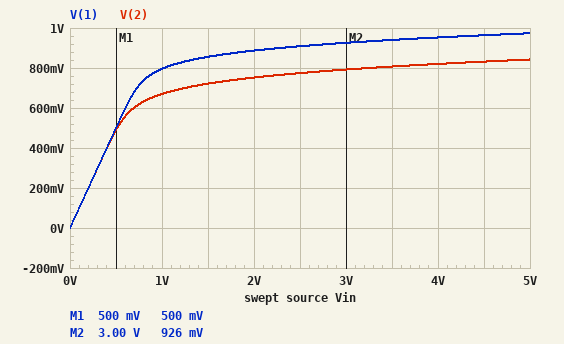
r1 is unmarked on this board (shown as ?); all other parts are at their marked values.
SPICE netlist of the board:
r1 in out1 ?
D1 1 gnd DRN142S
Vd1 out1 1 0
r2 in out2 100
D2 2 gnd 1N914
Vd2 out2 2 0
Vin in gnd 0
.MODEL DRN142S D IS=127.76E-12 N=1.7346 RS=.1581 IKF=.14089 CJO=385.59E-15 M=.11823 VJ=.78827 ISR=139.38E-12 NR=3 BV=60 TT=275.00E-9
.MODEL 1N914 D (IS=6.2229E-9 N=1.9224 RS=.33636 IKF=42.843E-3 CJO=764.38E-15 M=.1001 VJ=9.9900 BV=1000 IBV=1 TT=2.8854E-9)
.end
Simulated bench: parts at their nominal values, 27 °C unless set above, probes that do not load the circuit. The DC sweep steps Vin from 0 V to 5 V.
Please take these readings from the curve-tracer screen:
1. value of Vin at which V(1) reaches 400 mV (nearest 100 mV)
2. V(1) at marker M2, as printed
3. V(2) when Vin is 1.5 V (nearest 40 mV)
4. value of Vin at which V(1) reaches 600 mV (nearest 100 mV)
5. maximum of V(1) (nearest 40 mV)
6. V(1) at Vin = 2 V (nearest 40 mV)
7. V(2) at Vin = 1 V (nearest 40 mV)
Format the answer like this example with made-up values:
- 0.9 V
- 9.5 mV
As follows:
- 400 mV
- 926 mV
- 720 mV
- 600 mV
- 960 mV
- 880 mV
- 680 mV
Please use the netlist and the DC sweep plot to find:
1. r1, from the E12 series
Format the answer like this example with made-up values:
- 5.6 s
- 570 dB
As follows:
- 39 Ω
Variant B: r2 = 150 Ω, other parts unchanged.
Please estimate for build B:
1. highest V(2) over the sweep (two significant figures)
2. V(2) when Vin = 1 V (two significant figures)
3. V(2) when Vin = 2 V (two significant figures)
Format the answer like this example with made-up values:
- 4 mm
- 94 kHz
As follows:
- 810 mV
- 650 mV
- 730 mV
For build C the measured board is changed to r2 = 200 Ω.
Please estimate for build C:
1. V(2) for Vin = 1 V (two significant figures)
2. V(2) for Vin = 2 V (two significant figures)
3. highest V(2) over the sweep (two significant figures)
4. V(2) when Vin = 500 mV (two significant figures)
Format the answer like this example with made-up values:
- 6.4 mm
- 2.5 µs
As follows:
- 640 mV
- 710 mV
- 790 mV
- 480 mV
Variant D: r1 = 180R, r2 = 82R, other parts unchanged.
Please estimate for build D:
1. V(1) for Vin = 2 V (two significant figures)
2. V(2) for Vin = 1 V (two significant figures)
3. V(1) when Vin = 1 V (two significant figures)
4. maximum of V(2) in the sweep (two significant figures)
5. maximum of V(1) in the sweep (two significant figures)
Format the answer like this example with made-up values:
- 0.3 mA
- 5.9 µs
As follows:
- 810 mV
- 680 mV
- 730 mV
- 860 mV
- 870 mV
